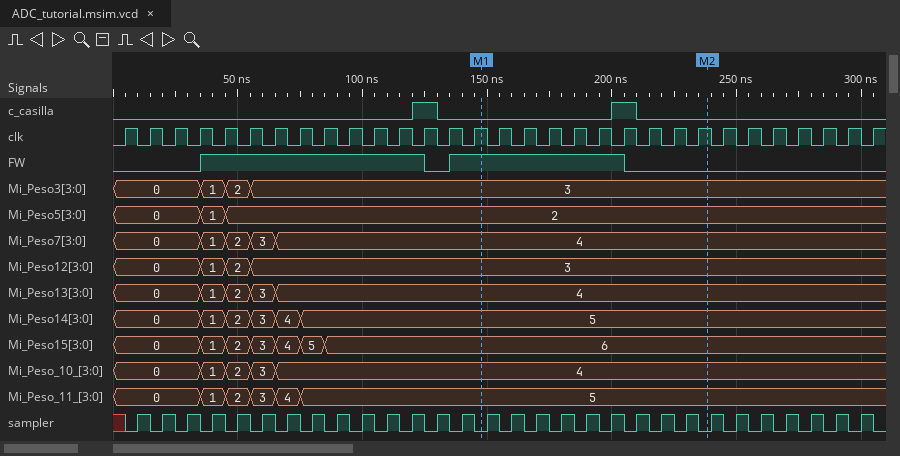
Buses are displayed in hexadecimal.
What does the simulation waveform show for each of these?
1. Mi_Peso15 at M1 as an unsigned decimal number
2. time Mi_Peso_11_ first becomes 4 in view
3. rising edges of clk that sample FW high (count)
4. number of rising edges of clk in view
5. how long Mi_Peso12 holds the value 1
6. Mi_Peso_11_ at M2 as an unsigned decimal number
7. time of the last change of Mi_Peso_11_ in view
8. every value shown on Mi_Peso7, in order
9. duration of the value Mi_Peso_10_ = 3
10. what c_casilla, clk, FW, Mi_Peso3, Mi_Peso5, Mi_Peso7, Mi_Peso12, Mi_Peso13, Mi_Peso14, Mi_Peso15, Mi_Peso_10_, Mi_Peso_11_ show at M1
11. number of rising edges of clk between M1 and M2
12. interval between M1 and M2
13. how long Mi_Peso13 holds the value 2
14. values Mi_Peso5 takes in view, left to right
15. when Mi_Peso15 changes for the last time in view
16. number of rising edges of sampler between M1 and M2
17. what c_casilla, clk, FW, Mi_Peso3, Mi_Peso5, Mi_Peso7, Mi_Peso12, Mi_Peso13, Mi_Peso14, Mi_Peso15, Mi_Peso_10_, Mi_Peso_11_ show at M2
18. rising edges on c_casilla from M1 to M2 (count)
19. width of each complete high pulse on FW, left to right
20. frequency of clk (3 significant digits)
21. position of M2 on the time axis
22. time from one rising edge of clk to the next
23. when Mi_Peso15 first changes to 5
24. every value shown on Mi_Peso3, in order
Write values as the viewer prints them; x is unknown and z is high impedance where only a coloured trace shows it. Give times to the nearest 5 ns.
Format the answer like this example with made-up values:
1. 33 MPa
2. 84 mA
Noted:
1. 6
2. 65 ns
3. 16
4. 31
5. 10 ns
6. 5
7. 75 ns
8. 0, 1, 2, 3, 4
9. 10 ns
10. c_casilla=0, clk=1, FW=1, Mi_Peso3=3, Mi_Peso5=2, Mi_Peso7=4, Mi_Peso12=3, Mi_Peso13=4, Mi_Peso14=5, Mi_Peso15=6, Mi_Peso_10_=4, Mi_Peso_11_=5
11. 9
12. 90 ns
13. 10 ns
14. 0, 1, 2
15. 85 ns
16. 9
17. c_casilla=0, clk=1, FW=0, Mi_Peso3=3, Mi_Peso5=2, Mi_Peso7=4, Mi_Peso12=3, Mi_Peso13=4, Mi_Peso14=5, Mi_Peso15=6, Mi_Peso_10_=4, Mi_Peso_11_=5
18. 1
19. 90 ns, 70 ns
20. 100 MHz
21. 240 ns
22. 10 ns
23. 75 ns
24. 0, 1, 2, 3
